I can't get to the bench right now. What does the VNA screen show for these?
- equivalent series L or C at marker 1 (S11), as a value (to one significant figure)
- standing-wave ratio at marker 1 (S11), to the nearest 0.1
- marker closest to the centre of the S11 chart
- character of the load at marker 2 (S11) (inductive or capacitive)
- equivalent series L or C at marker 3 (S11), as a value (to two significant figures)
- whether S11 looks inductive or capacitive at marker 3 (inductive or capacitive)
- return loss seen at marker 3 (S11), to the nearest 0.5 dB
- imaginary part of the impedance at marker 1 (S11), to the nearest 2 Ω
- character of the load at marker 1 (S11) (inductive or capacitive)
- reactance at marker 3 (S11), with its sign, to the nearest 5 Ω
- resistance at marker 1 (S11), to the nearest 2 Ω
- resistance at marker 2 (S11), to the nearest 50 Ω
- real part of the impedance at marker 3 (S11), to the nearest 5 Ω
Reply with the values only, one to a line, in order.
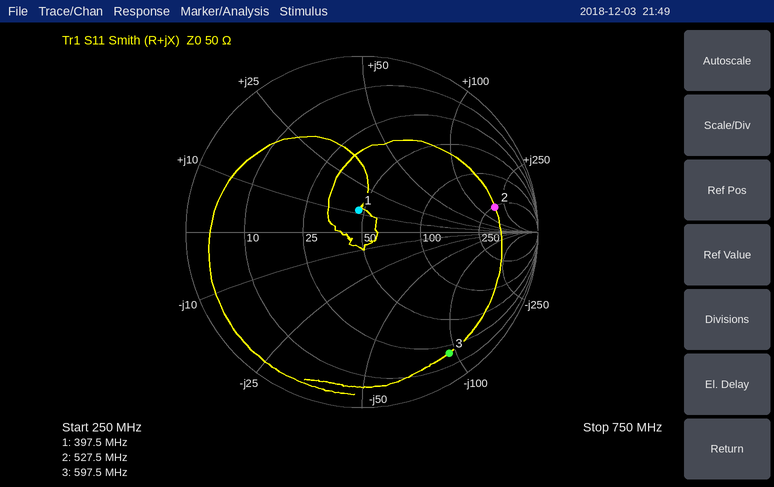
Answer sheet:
5 nH
1.3
marker 1
inductive
2.8 pF
capacitive
1.5 dB
+12 Ω
inductive
-95 Ω
46 Ω
250 Ω
20 Ω
